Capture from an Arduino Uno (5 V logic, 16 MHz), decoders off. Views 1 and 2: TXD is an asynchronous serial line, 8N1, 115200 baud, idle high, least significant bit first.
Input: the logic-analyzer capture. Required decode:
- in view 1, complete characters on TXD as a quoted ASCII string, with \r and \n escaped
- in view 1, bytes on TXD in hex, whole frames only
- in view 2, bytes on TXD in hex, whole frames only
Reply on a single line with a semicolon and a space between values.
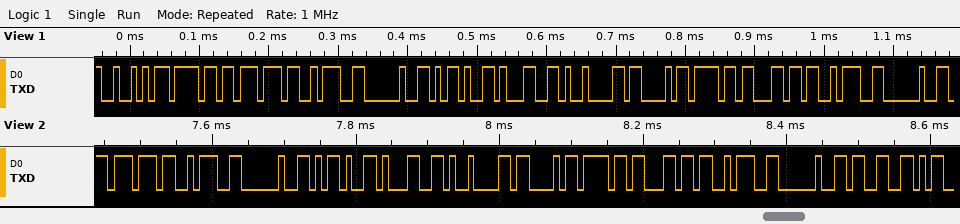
"Row: -1\tCol: "; 52 6F 77 3A 20 2D 31 09 43 6F 6C 3A 20; 0x77 0x3A 0x20 0x2D 0x31 0x09 0x43 0x6F 0x6C 0x3A 0x20 0x33
